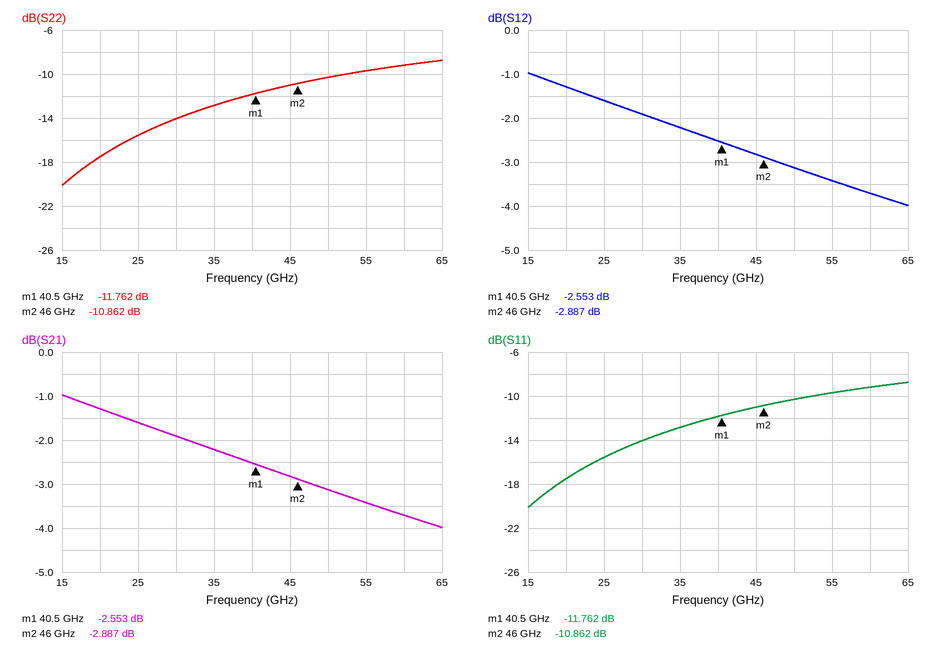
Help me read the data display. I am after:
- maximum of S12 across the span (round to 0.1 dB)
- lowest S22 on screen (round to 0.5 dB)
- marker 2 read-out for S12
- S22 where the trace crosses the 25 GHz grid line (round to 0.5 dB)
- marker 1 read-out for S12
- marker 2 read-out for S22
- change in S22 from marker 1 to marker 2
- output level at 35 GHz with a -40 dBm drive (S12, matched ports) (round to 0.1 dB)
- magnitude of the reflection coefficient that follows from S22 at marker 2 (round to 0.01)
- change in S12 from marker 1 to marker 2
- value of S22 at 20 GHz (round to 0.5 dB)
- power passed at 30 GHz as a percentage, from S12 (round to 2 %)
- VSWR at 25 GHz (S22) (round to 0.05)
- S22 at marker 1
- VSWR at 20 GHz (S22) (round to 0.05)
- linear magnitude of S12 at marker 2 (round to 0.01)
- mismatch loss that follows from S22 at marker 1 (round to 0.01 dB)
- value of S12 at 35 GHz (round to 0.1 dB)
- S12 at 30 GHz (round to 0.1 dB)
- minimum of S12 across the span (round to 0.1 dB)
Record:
-1.0 dB
-20.0 dB
-2.887 dB
-15.5 dB
-2.553 dB
-10.862 dB
0.900 dB
-42.2 dBm
0.29
-0.334 dB
-17.5 dB
64 %
1.40
-11.762 dB
1.30
0.72
0.30 dB
-2.2 dB
-1.9 dB
-4.0 dB
